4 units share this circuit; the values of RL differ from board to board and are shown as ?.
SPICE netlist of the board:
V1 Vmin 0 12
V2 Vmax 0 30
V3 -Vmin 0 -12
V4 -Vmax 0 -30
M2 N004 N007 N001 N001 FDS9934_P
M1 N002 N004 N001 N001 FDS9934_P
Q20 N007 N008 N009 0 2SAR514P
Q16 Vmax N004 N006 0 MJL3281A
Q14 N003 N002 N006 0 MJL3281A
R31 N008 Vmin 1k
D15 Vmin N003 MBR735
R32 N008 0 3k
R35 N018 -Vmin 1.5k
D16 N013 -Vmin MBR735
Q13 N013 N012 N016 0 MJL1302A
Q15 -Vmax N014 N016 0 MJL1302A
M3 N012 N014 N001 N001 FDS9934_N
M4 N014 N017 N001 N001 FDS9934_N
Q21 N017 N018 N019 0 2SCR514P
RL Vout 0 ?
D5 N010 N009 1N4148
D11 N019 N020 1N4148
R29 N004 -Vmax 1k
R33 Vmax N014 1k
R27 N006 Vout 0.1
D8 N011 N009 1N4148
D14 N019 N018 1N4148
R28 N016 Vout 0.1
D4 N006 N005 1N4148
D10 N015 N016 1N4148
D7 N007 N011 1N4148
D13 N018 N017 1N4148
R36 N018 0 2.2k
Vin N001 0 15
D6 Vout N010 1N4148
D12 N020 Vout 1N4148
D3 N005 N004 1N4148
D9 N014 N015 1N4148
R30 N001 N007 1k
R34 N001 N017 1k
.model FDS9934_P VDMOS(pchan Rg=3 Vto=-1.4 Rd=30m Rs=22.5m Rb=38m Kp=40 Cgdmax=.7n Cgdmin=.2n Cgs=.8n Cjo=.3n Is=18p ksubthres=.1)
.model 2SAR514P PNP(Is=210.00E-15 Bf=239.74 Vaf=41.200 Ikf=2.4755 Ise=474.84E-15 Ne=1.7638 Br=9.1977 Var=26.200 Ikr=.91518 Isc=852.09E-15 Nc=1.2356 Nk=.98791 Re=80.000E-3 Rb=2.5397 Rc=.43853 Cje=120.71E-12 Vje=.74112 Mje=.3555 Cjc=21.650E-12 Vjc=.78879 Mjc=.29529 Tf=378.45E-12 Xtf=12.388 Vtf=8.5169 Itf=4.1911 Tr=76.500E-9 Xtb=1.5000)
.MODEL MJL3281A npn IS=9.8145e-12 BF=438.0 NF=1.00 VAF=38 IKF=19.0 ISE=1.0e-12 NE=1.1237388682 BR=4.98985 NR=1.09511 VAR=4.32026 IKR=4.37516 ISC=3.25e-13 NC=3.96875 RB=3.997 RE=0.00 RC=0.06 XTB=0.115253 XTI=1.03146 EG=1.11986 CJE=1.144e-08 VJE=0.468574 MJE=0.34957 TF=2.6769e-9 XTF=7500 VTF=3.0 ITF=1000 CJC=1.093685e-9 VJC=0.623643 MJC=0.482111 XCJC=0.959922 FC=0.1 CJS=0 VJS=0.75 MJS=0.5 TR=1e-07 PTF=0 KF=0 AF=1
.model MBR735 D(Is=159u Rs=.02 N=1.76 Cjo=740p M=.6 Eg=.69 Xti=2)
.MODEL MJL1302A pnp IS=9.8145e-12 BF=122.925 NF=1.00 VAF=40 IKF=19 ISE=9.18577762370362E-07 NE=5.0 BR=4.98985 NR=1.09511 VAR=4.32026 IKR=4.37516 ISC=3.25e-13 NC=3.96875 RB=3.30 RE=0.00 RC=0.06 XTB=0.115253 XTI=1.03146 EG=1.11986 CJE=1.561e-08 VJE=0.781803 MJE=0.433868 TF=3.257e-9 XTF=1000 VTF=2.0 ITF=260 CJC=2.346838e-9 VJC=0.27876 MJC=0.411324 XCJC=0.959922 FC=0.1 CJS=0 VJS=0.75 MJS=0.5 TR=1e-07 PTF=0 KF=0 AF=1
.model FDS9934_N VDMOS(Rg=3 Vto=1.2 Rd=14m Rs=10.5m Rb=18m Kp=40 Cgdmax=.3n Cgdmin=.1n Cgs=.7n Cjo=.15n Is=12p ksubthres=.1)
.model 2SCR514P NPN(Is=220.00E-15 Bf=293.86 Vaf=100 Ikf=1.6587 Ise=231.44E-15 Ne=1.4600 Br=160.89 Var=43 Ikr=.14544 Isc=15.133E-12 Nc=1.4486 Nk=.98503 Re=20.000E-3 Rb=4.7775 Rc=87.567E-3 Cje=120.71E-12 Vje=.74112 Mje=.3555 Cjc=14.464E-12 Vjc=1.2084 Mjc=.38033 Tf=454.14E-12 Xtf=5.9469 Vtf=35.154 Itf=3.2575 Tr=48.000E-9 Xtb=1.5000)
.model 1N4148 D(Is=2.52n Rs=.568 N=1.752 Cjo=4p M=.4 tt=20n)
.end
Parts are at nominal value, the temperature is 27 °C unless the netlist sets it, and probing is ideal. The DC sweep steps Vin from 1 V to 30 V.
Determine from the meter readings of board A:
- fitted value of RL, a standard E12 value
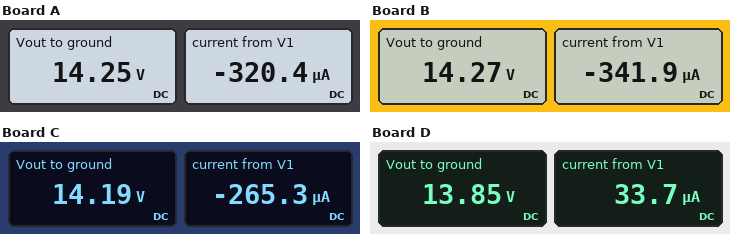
18 Ω
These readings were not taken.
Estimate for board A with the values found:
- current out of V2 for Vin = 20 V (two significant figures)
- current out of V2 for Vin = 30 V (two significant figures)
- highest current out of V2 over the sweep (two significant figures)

1.1 A
1.6 A
1.6 A
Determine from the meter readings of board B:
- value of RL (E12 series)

22 Ω
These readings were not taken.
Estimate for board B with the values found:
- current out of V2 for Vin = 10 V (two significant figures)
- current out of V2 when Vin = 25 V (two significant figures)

19 mA
1.1 A
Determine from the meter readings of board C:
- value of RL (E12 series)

12 Ω
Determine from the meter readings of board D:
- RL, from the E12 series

3.9 Ω
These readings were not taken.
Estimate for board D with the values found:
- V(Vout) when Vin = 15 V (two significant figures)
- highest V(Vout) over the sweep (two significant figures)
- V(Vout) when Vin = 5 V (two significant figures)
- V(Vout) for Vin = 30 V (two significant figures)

14 V
28 V
4.2 V
28 V
